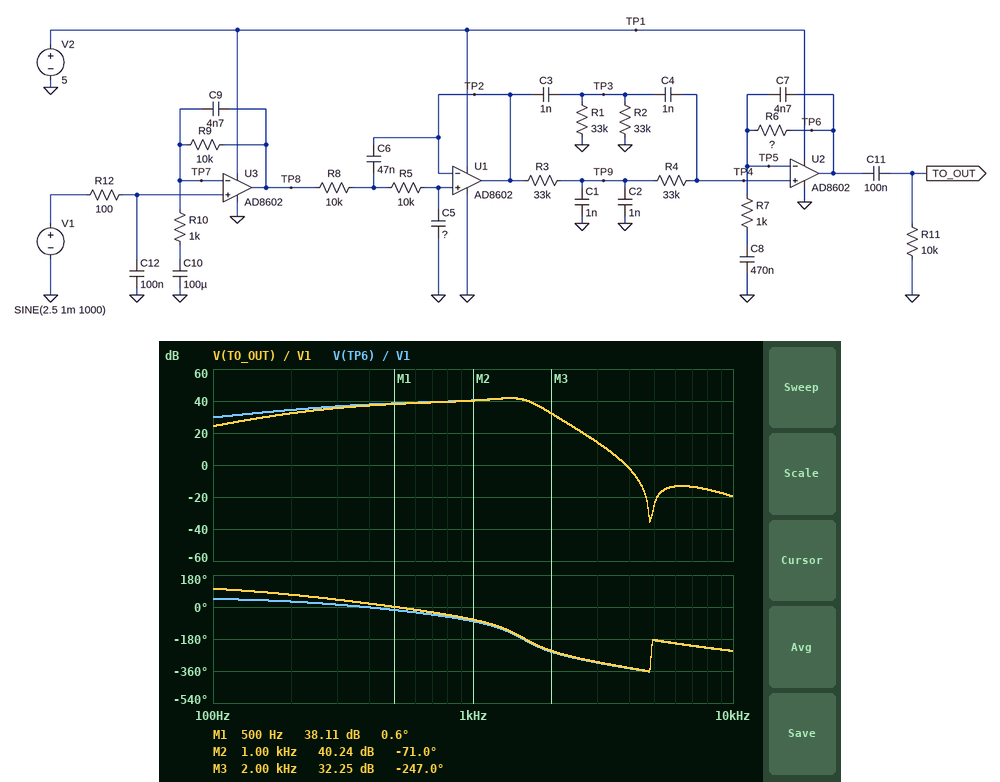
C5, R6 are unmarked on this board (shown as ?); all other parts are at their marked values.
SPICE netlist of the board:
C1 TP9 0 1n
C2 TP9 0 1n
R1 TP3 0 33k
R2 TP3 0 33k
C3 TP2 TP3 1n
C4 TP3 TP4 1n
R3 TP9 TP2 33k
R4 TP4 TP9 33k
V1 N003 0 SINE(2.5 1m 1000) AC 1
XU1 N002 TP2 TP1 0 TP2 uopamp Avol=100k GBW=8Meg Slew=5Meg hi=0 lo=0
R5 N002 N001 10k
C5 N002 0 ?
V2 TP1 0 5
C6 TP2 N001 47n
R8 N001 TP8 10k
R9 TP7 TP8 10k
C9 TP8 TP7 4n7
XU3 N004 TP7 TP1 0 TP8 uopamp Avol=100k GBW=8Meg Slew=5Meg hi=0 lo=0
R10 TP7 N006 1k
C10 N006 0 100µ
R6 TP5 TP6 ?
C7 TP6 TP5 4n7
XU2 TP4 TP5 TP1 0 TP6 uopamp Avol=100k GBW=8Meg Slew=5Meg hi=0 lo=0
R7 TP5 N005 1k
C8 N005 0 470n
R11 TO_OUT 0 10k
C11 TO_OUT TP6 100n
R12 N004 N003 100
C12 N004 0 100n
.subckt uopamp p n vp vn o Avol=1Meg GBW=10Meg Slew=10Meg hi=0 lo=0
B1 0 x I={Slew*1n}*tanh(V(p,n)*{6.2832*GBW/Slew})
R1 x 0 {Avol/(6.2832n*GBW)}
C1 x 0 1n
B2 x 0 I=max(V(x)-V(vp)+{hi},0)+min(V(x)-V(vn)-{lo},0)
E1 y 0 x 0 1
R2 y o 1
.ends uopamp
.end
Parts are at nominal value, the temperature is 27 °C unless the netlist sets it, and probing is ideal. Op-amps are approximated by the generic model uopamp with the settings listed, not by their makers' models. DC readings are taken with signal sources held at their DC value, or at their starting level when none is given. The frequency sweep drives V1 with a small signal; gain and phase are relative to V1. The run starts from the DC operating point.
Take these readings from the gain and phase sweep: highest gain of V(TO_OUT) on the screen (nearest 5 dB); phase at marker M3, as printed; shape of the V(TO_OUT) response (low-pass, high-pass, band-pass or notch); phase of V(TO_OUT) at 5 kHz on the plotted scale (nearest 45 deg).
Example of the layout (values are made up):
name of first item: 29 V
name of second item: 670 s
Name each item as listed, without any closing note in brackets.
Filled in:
highest gain of V(TO_OUT) on the screen: 40 dB
phase at marker M3, as printed: -247.0 deg
shape of the V(TO_OUT) response: band-pass
phase of V(TO_OUT) at 5 kHz on the plotted scale: -180 deg
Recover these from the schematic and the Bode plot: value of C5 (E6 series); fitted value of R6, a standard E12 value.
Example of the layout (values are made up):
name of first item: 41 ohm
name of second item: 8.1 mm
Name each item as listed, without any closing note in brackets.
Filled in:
value of C5: 2.2 nF
fitted value of R6, a standard E12 value: 8.2 kΩ
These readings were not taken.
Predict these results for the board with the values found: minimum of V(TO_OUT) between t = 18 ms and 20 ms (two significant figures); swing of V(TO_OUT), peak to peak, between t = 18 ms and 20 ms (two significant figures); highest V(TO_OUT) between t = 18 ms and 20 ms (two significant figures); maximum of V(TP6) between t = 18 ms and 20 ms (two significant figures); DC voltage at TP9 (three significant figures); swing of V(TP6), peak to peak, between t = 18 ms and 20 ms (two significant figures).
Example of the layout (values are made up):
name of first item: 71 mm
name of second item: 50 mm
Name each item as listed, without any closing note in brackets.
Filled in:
minimum of V(TO_OUT) between t = 18 ms and 20 ms: -100 mV
swing of V(TO_OUT), peak to peak, between t = 18 ms and 20 ms: 210 mV
highest V(TO_OUT) between t = 18 ms and 20 ms: 100 mV
maximum of V(TP6) between t = 18 ms and 20 ms: 2.6 V
DC voltage at TP9: 2.50 V
swing of V(TP6), peak to peak, between t = 18 ms and 20 ms: 210 mV
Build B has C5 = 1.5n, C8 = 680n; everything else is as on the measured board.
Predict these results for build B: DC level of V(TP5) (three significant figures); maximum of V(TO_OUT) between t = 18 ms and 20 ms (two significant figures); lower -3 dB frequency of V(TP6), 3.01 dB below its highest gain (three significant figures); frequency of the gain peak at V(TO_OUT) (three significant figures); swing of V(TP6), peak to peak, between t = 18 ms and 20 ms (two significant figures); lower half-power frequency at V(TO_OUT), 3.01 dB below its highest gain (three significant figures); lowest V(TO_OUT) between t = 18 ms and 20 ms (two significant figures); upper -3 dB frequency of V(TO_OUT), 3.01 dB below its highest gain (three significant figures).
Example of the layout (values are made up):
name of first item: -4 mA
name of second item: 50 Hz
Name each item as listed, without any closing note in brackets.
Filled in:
DC level of V(TP5): 2.50 V
maximum of V(TO_OUT) between t = 18 ms and 20 ms: 92 mV
lower -3 dB frequency of V(TP6), 3.01 dB below its highest gain: 340 Hz
frequency of the gain peak at V(TO_OUT): 1.73 kHz
swing of V(TP6), peak to peak, between t = 18 ms and 20 ms: 190 mV
lower half-power frequency at V(TO_OUT), 3.01 dB below its highest gain: 438 Hz
lowest V(TO_OUT) between t = 18 ms and 20 ms: -92 mV
upper -3 dB frequency of V(TO_OUT), 3.01 dB below its highest gain: 2.03 kHz
